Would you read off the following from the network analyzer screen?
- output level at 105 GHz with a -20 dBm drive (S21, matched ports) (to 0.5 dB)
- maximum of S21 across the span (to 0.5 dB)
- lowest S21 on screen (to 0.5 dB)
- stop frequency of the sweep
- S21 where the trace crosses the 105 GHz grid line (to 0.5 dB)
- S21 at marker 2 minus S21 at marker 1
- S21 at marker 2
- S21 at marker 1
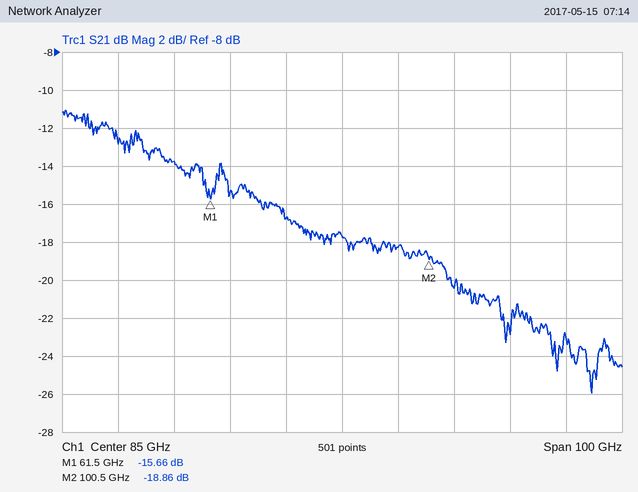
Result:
-40.5 dBm
-11.0 dB
-26.0 dB
135 GHz
-20.5 dB
-3.20 dB
-18.86 dB
-15.66 dB
